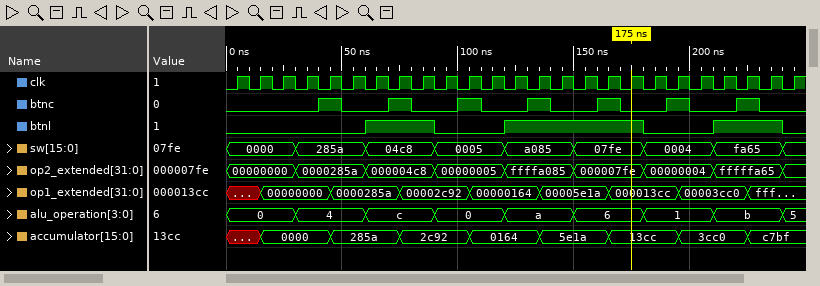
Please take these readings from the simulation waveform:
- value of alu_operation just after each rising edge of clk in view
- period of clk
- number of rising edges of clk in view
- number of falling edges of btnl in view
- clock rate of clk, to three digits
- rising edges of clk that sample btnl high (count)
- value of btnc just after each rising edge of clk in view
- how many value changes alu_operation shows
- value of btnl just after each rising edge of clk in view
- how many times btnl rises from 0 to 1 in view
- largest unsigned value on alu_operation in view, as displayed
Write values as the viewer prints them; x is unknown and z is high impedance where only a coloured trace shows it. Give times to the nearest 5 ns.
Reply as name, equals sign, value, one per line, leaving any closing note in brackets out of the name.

value of alu_operation just after each rising edge of clk in view = 0, 0, 0, 4, 4, 4, c, c, c, 0, 0, 0, a, a, a, 6, 6, 6, 1, 1, 1, b, b, b, 5
period of clk = 10 ns
number of rising edges of clk in view = 25
number of falling edges of btnl in view = 3
clock rate of clk, to three digits = 100 MHz
rising edges of clk that sample btnl high = 12
value of btnc just after each rising edge of clk in view = 0 0 0 0 1 0 0 1 0 0 1 0 0 1 0 0 1 0 0 1 0 0 1 0 0
how many value changes alu_operation shows = 8
value of btnl just after each rising edge of clk in view = 0 0 0 0 0 0 1 1 1 0 0 0 1 1 1 1 1 1 0 0 0 1 1 1 0
how many times btnl rises from 0 to 1 in view = 3
largest unsigned value on alu_operation in view, as displayed = c
